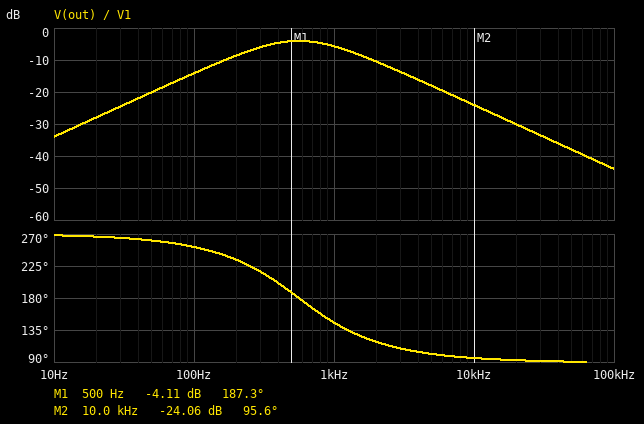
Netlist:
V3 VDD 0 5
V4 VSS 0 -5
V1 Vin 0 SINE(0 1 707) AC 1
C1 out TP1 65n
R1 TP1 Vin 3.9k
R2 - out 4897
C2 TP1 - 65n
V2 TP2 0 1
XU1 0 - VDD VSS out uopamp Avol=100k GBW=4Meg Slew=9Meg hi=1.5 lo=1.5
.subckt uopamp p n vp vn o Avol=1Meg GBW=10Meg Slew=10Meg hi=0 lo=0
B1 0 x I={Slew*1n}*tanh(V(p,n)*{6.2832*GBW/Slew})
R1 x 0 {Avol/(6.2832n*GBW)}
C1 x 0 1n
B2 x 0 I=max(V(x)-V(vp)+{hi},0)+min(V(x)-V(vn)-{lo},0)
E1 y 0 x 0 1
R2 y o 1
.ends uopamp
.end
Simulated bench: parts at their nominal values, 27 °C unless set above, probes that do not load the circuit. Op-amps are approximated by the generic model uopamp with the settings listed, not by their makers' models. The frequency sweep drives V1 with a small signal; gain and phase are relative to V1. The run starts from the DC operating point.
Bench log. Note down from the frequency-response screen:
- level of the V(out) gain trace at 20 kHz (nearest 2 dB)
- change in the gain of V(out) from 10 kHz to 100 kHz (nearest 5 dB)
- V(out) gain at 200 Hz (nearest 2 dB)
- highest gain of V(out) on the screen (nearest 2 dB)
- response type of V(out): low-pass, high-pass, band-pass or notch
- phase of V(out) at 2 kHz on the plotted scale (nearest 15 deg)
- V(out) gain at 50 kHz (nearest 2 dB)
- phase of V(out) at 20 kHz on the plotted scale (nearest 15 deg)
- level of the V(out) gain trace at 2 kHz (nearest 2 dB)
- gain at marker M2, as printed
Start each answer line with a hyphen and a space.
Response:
- -30 dB
- -20 dB
- -8 dB
- -4 dB
- band-pass
- 120 deg
- -38 dB
- 90 deg
- -10 dB
- -24.06 dB
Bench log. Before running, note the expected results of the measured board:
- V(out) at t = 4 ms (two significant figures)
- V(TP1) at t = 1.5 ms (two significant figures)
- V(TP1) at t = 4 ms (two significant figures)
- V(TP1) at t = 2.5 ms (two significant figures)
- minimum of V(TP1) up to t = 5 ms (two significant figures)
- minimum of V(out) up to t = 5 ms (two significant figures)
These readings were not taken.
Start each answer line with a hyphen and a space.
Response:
- 590 mV
- -420 mV
- -99 mV
- 63 mV
- -430 mV
- -610 mV
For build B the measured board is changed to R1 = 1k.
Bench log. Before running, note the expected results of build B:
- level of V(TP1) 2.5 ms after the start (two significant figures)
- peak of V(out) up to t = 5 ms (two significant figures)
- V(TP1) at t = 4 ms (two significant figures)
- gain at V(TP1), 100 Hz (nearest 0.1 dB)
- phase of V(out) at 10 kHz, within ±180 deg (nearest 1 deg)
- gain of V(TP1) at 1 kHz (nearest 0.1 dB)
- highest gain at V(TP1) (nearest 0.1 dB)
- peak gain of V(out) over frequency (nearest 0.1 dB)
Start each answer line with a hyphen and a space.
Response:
- -950 mV
- 1.7 V
- -1.2 V
- 0 dB
- 96 deg
- 1.5 dB
- 1.9 dB
- 7.8 dB
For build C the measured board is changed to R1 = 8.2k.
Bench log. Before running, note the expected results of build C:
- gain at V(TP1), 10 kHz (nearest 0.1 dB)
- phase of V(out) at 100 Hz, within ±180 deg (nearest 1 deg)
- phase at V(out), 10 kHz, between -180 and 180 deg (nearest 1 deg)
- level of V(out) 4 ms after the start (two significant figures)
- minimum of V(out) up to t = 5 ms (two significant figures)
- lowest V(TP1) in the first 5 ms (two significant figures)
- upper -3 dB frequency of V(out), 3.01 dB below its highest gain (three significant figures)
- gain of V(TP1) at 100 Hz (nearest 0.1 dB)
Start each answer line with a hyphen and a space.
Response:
- -57.0 dB
- -126 deg
- 96 deg
- 270 mV
- -270 mV
- -190 mV
- 1.13 kHz
- -1.2 dB
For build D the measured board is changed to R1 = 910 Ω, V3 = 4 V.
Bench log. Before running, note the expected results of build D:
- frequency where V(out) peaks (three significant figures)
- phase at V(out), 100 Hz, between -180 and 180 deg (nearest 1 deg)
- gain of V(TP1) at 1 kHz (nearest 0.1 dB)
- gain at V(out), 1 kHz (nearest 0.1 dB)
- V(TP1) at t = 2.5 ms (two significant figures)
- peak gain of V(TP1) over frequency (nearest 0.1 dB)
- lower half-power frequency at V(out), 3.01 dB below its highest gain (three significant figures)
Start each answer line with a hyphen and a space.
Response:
- 1.16 kHz
- -94 deg
- 2.1 dB
- 8.1 dB
- -1.0 V
- 2.2 dB
- 763 Hz
